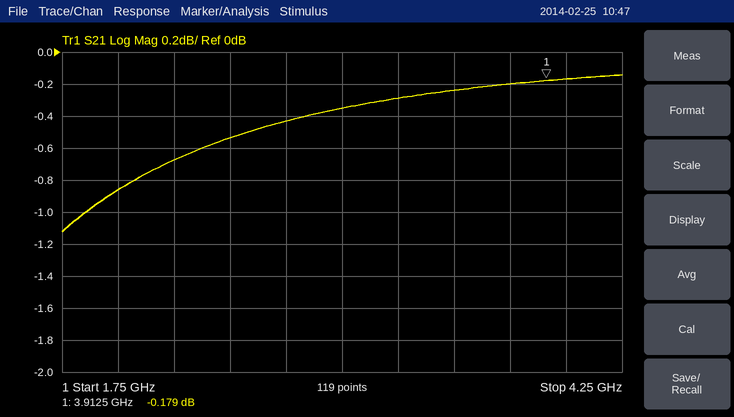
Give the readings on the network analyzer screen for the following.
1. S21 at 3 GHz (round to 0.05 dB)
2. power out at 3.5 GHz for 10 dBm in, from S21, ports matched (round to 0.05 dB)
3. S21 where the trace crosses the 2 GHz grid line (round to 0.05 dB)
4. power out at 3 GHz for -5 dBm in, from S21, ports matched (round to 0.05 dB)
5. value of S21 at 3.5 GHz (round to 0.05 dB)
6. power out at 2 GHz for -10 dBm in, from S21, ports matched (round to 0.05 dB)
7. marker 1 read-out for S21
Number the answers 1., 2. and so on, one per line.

1. -0.35 dB
2. 9.75 dBm
3. -0.85 dB
4. -5.35 dBm
5. -0.25 dB
6. -10.85 dBm
7. -0.179 dB
